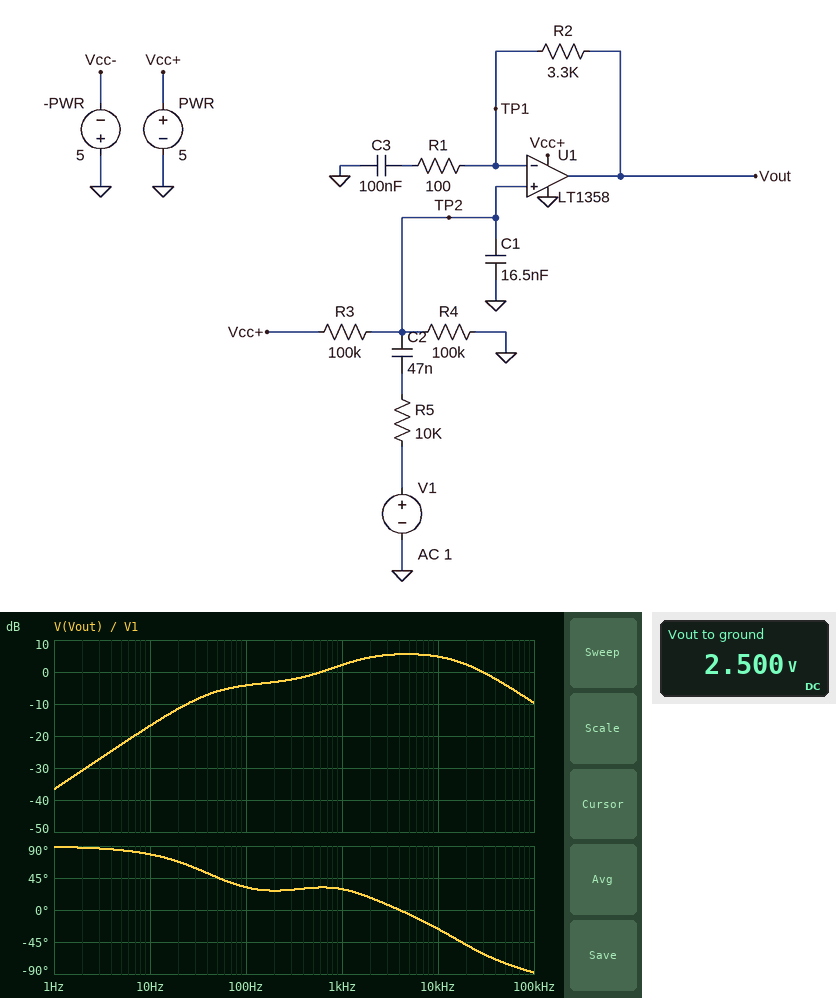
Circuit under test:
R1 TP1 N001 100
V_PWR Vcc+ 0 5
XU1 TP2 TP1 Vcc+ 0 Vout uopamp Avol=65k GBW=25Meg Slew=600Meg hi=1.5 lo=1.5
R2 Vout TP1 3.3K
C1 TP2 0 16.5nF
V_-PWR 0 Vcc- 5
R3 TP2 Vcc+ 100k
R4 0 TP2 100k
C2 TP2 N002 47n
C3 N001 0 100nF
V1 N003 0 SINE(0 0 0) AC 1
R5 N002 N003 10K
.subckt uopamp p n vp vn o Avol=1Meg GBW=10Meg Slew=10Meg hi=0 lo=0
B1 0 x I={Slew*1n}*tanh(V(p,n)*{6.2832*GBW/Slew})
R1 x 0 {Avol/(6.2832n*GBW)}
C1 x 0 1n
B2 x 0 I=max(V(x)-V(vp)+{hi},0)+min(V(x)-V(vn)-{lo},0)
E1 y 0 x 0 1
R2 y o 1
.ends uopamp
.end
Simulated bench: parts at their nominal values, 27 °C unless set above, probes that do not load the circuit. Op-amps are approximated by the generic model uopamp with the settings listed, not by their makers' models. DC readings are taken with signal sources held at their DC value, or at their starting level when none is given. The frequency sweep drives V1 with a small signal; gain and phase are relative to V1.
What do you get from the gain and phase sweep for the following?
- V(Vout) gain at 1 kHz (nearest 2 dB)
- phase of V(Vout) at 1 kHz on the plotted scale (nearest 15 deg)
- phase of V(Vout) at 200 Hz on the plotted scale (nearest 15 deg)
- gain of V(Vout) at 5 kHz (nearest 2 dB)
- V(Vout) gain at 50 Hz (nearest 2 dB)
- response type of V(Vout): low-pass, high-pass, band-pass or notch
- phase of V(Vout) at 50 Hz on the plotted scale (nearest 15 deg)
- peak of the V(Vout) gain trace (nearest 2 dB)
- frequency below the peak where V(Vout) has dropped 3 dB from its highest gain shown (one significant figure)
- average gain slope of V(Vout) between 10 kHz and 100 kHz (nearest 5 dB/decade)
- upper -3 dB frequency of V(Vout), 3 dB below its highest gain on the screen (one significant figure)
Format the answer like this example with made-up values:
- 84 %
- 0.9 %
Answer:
- 2 dB
- 30 deg
- 30 deg
- 6 dB
- -6 dB
- band-pass
- 45 deg
- 6 dB
- 1 kHz
- -15 dB/decade
- 20 kHz
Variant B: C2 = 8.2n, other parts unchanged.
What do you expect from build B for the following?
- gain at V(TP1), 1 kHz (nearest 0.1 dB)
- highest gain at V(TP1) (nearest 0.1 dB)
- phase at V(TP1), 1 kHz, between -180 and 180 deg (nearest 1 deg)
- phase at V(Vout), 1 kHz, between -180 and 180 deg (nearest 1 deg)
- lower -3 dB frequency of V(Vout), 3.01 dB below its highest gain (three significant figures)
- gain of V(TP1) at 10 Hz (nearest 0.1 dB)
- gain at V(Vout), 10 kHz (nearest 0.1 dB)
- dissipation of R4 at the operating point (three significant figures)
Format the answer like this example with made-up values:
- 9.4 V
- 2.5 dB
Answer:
- -10.3 dB
- -10.1 dB
- -11 deg
- 50 deg
- 2.18 kHz
- -31.8 dB
- 4.5 dB
- 62.5 µW
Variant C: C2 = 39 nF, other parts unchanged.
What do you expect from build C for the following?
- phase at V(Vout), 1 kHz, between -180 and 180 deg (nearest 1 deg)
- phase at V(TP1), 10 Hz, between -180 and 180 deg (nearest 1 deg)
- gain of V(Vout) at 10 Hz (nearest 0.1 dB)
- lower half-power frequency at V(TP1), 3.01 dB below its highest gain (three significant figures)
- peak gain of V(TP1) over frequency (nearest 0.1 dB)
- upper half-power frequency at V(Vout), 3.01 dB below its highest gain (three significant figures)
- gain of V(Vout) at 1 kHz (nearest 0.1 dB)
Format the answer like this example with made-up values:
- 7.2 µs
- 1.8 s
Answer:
- 31 deg
- 79 deg
- -18.4 dB
- 48.8 Hz
- -4.2 dB
- 18.9 kHz
- 1.9 dB
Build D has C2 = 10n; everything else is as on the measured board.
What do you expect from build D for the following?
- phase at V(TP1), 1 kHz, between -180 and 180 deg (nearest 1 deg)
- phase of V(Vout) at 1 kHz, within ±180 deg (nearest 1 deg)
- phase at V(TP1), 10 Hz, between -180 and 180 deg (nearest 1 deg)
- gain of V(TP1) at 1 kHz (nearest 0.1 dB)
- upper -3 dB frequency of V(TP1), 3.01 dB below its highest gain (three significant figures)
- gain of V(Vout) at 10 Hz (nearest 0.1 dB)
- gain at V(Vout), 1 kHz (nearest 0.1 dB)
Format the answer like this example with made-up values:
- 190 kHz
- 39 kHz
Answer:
- -14 deg
- 47 deg
- 85 deg
- -9.4 dB
- 2.86 kHz
- -30.1 dB
- -1.9 dB
